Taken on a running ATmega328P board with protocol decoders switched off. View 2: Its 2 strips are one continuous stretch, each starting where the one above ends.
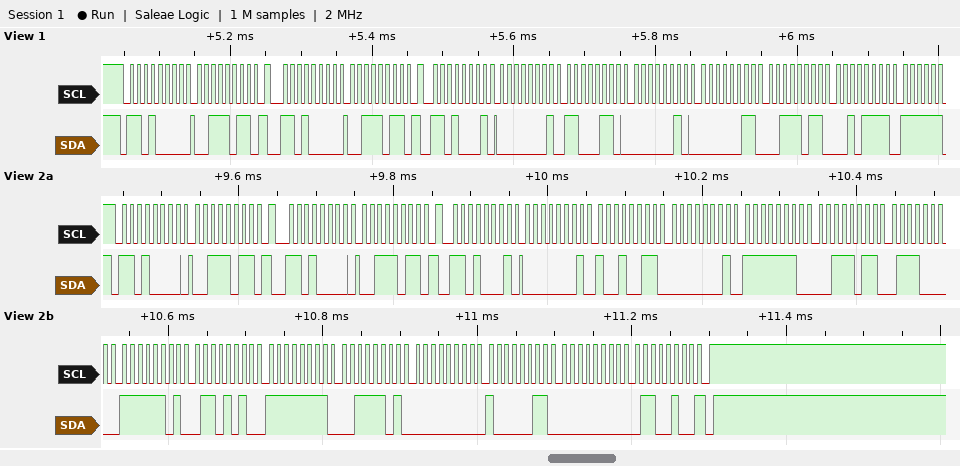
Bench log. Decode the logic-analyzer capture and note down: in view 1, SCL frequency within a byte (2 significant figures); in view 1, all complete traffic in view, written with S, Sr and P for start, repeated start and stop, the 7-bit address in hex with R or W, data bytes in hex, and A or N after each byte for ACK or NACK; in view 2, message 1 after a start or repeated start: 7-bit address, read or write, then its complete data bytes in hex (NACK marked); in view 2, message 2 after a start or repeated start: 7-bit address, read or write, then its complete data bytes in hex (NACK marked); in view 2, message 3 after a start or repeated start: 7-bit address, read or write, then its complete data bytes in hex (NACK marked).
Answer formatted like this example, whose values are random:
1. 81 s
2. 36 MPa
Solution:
1. 100 kHz
2. S 68W A 3B A Sr 68W A 3B A Sr 68R A 01 A C6 A 02 A 03 A 3B A 2F A
3. 0x68 write: 3B
4. 0x68 write: 3B
5. 0x68 read: 01 93 01 FE 3B 70 FD 6A FF 3D 00 83 00 64 NACK
